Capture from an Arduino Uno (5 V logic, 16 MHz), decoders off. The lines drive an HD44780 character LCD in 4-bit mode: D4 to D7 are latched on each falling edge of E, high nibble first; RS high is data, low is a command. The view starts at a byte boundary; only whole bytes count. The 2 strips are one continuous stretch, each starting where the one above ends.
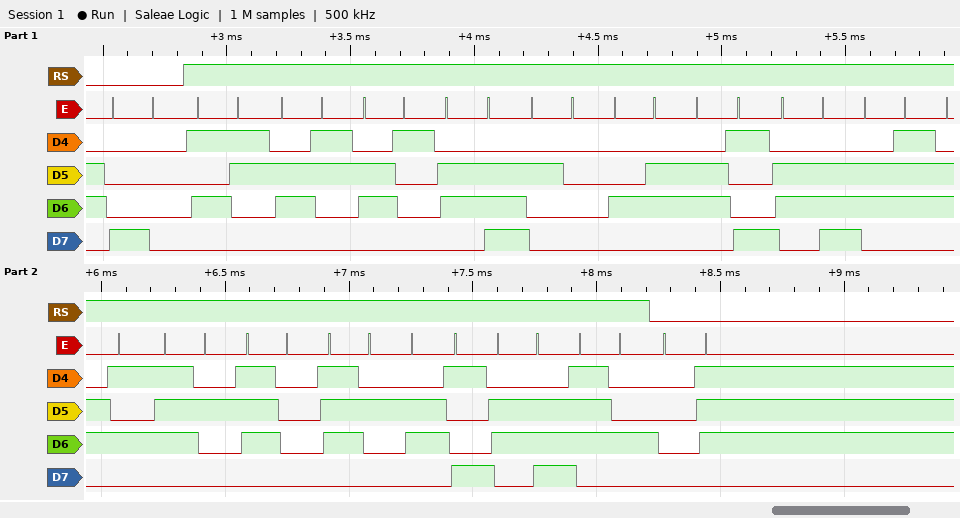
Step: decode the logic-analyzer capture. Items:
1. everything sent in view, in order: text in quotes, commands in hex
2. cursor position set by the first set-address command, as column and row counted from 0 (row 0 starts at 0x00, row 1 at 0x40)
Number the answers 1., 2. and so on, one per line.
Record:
1. 0x80 "Scan Fingerprint" 0x07
2. column 0, row 0
